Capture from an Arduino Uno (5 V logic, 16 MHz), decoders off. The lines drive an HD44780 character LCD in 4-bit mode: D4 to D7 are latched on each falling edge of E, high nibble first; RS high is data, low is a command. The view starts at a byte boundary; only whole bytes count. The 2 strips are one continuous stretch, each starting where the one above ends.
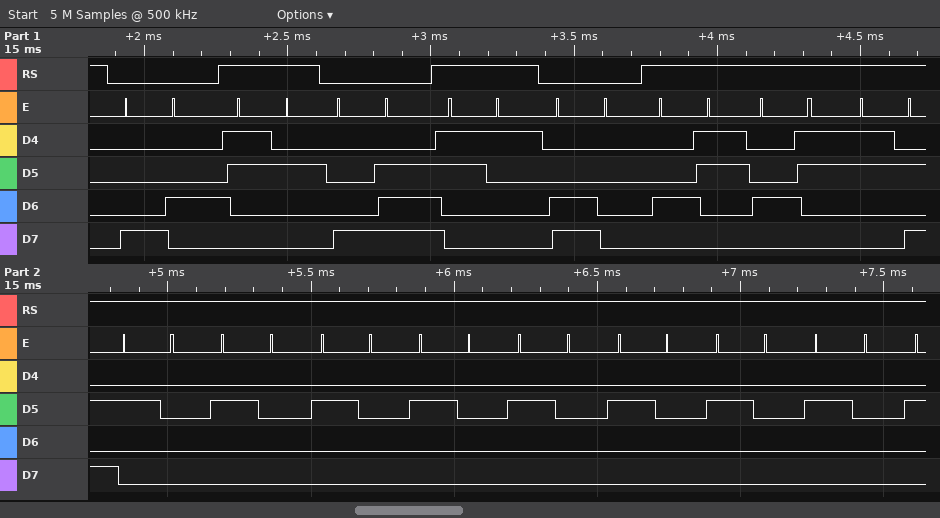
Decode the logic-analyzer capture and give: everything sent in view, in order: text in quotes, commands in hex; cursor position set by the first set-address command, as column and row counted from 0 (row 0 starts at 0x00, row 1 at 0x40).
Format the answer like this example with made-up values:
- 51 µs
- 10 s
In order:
- 0x84 "2" 0x8E "1" 0xC0 "CC:        "
- column 4, row 0
